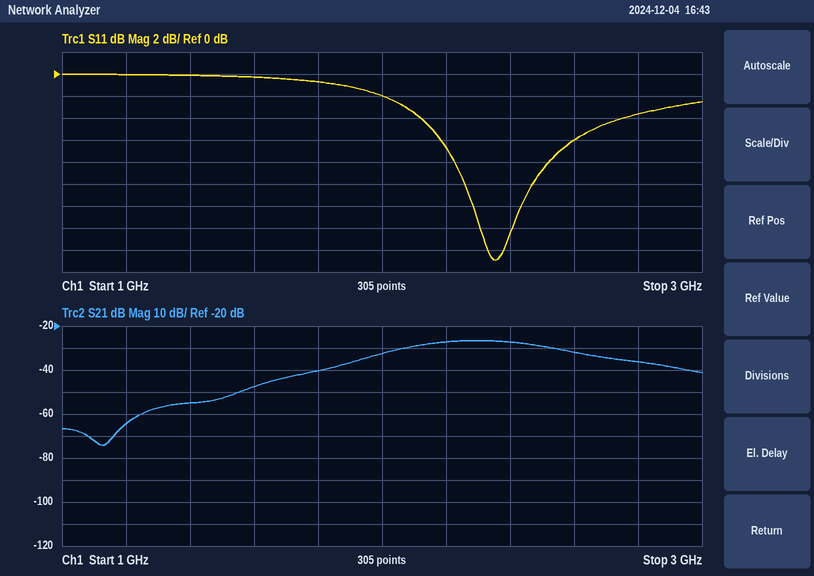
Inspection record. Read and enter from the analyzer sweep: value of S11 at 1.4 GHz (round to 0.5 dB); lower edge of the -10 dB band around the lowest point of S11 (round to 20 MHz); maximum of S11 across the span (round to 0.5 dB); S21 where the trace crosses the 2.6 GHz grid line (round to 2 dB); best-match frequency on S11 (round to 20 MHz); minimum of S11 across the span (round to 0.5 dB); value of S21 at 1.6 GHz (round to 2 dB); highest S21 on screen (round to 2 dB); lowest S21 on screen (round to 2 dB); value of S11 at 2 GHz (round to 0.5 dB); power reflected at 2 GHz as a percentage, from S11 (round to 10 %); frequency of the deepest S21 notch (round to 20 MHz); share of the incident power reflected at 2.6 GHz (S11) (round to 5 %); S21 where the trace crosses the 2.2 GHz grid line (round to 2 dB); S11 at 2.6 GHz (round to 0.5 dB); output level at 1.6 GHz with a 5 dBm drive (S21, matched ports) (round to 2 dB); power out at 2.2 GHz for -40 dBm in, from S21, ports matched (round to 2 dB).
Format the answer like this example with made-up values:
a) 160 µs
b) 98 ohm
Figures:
a) 0.0 dB
b) 2.26 GHz
c) 0.0 dB
d) -32 dB
e) 2.36 GHz
f) -17.0 dB
g) -48 dB
h) -26 dB
i) -74 dB
j) -2.0 dB
k) 60 %
l) 1.12 GHz
m) 25 %
n) -28 dB
o) -6.0 dB
p) -42 dBm
q) -68 dBm
